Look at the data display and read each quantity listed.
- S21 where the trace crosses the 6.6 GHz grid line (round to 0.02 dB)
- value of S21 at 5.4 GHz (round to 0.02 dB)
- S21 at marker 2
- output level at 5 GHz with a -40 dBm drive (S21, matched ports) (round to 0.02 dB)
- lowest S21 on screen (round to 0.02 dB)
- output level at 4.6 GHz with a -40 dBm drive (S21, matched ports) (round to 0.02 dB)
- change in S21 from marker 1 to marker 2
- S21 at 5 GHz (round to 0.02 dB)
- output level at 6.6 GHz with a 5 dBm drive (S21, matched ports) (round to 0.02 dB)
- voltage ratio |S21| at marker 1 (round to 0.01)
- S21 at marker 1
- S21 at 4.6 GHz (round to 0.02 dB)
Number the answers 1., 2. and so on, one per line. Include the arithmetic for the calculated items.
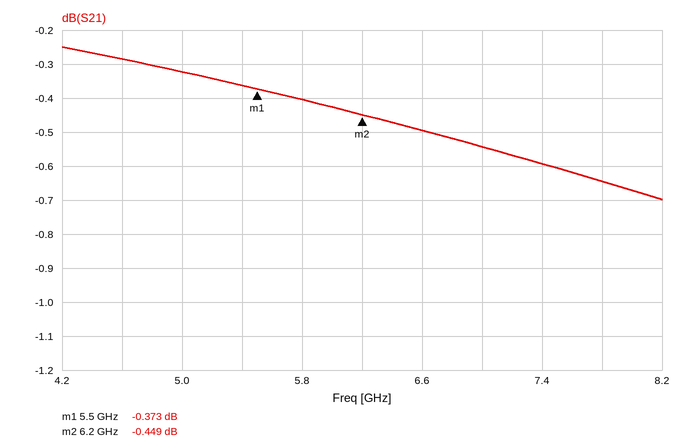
1. -0.50 dB
2. -0.36 dB
3. -0.449 dB
4. -40 dBm + (-0.32 dB) = -40.32 dBm
5. -0.70 dB
6. -40 dBm + (-0.28 dB) = -40.28 dBm
7. -0.449 − (-0.373) = -0.076 dB
8. -0.32 dB
9. 5 dBm + (-0.50 dB) = 4.50 dBm
10. 10^(-0.373/20) ≈ 0.96
11. -0.373 dB
12. -0.28 dB
